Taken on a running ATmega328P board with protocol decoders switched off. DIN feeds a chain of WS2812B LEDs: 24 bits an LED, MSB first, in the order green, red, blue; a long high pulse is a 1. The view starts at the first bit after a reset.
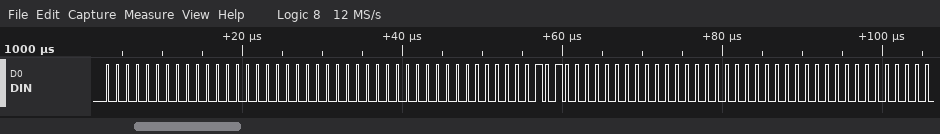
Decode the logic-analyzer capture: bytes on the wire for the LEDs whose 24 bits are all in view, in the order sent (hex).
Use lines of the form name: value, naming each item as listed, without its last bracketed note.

bytes on the wire for the LEDs whose 24 bits are all in view, in the order sent: 00 00 00 00 00 14 00 00 00
